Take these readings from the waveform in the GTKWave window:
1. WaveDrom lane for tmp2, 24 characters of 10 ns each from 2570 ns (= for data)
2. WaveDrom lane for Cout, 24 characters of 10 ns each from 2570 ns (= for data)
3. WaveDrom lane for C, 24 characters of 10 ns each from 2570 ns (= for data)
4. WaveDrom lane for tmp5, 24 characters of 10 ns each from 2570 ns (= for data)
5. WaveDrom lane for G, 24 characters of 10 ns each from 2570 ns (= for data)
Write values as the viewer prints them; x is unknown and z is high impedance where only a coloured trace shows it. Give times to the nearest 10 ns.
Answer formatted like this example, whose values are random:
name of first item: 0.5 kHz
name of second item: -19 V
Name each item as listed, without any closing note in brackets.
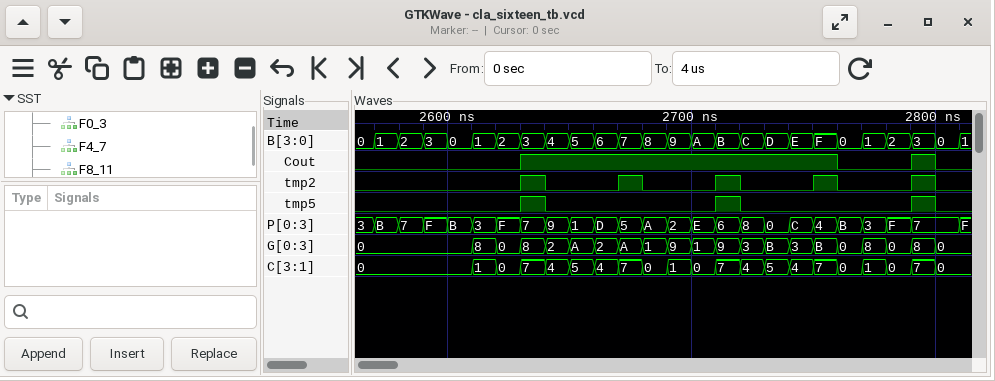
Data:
WaveDrom lane for tmp2, 24 characters of 10 ns each from 2570 ns: {name: 'tmp2', wave: '0.....10..10..10..10..10'}
WaveDrom lane for Cout, 24 characters of 10 ns each from 2570 ns: {name: 'Cout', wave: '0.....1............0..10'}
WaveDrom lane for C, 24 characters of 10 ns each from 2570 ns: {name: 'C', wave: '=...====================', data: '0 1 0 7 4 5 4 7 0 1 0 7 4 5 4 7 0 1 0 7 0'}
WaveDrom lane for tmp5, 24 characters of 10 ns each from 2570 ns: {name: 'tmp5', wave: '0.....10......10......10'}
WaveDrom lane for G, 24 characters of 10 ns each from 2570 ns: {name: 'G', wave: '=...====================', data: '0 8 0 8 2 A 2 A 1 9 1 9 3 B 3 B 0 8 0 8 0'}
